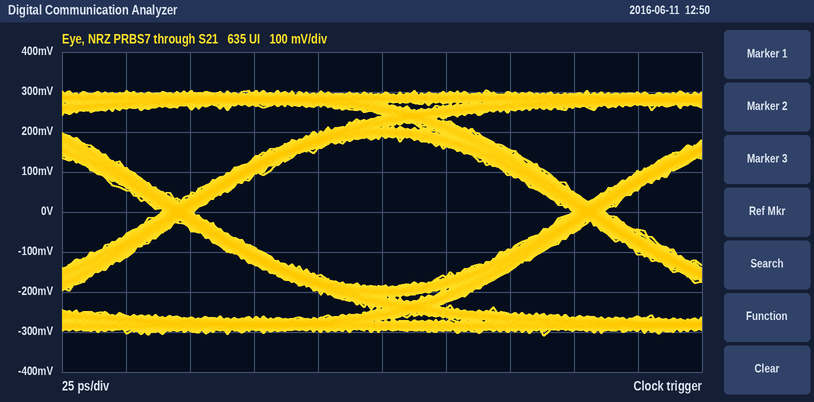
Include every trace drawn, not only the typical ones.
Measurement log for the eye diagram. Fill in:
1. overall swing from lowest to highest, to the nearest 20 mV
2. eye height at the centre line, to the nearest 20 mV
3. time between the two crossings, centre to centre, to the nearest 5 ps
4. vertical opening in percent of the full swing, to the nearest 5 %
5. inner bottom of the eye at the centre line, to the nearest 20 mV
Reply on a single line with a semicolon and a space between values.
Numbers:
620 mV; 380 mV; 160 ps; 60 %; -180 mV
